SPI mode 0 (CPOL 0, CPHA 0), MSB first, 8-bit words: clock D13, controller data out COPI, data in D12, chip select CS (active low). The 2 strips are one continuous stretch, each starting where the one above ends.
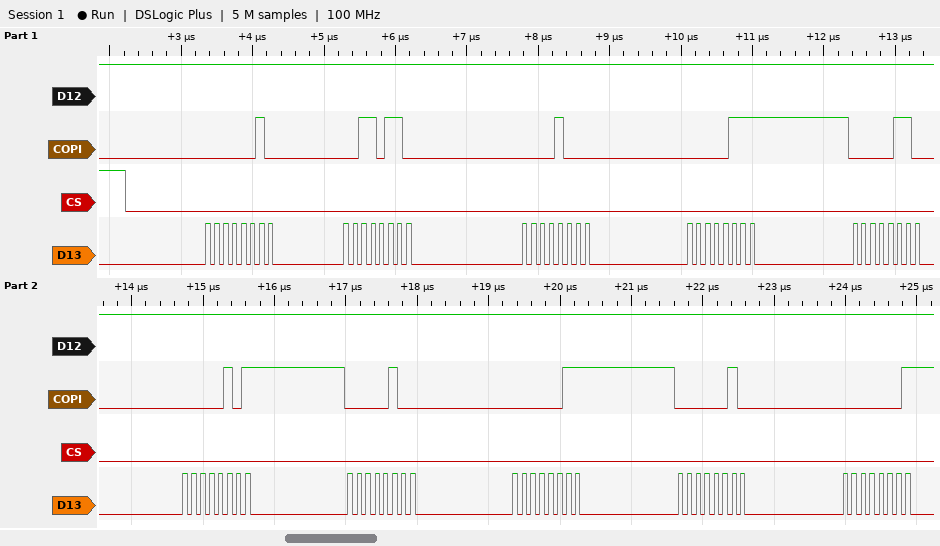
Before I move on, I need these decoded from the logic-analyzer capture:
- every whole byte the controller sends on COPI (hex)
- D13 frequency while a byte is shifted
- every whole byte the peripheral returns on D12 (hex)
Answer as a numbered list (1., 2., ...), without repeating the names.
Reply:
1. 02 36 08 07 06 05 04 03 02 01
2. 8 MHz
3. FF FF FF FF FF FF FF FF FF FF
